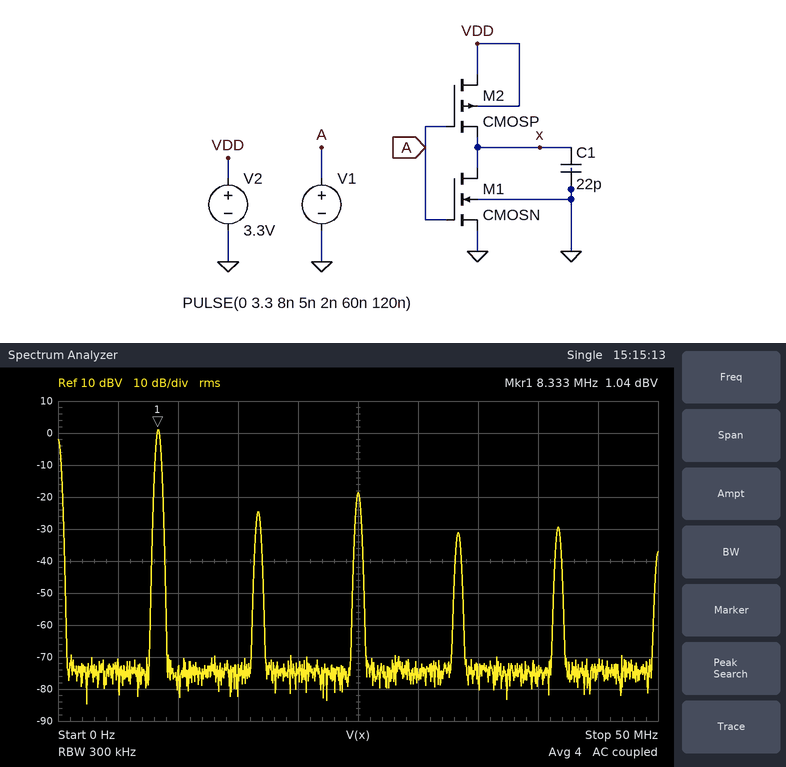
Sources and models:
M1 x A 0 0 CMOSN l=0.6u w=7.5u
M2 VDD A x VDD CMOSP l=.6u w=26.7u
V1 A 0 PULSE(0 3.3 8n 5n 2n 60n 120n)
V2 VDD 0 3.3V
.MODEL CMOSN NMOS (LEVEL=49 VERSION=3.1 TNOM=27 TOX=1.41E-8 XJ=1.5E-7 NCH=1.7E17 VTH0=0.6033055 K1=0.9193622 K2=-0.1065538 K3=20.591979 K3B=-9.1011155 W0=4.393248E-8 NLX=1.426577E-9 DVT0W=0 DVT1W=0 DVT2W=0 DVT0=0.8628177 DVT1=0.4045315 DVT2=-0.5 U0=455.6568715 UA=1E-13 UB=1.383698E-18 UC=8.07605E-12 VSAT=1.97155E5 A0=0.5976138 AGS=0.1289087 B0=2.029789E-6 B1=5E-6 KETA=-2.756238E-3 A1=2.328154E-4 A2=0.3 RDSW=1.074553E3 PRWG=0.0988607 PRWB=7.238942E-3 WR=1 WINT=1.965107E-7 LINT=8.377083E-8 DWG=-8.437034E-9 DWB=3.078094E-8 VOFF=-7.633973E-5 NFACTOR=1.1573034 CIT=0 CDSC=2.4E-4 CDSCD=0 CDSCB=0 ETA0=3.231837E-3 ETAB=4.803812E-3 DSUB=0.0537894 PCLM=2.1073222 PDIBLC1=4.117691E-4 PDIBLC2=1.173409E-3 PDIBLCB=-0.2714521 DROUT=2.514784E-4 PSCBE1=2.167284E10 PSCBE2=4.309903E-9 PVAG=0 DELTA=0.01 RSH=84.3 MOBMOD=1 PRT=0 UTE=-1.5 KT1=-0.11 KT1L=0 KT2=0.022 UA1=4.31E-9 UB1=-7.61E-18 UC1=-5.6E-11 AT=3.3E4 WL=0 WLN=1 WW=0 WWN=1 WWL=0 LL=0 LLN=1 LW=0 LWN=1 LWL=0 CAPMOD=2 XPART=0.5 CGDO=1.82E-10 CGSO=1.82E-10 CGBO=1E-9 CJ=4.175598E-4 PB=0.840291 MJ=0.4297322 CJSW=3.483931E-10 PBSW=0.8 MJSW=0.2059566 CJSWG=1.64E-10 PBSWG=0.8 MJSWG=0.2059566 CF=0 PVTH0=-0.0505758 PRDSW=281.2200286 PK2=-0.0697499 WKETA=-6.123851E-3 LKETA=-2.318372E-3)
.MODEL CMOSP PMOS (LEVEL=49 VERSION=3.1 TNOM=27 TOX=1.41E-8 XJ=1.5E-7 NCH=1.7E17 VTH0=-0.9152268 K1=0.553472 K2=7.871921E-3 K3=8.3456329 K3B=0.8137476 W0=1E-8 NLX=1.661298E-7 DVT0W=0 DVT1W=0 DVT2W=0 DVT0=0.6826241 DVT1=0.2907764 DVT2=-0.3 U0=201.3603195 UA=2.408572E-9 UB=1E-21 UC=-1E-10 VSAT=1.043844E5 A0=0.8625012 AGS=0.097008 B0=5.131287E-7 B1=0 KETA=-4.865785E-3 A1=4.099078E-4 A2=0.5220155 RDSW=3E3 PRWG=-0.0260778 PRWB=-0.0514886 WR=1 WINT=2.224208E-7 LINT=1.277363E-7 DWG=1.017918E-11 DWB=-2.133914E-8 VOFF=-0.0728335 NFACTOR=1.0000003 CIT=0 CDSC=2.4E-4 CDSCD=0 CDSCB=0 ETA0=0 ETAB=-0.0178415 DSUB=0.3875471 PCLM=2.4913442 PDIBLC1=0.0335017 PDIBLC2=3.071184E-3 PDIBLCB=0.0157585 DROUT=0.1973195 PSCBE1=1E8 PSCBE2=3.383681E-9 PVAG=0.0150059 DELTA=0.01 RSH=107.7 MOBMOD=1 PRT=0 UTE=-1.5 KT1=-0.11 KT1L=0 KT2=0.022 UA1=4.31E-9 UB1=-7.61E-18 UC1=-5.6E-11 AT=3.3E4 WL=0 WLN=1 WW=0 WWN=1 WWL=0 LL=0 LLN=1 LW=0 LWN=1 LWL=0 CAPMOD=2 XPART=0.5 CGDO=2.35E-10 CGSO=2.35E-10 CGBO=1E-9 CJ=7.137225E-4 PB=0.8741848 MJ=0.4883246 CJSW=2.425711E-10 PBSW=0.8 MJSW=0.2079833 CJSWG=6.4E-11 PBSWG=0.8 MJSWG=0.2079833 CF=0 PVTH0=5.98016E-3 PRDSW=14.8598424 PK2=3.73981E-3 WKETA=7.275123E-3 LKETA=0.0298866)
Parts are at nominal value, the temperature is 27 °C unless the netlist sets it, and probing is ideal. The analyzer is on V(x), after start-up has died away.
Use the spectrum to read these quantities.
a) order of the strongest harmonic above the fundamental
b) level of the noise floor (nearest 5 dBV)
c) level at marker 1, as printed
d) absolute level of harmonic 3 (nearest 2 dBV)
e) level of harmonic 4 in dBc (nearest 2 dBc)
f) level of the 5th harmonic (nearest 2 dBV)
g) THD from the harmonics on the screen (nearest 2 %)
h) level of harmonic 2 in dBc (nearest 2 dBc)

3
-75 dBV
1.04 dBV
-18 dBV
-32 dBc
-30 dBV
12 %
-26 dBc
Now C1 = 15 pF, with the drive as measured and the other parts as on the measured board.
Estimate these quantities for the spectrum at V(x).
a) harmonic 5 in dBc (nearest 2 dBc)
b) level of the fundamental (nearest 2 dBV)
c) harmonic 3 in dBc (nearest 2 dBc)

-28 dBc
2 dBV
-16 dBc
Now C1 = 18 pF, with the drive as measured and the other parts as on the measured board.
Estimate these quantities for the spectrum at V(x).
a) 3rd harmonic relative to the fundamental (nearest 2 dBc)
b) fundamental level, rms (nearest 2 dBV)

-18 dBc
2 dBV
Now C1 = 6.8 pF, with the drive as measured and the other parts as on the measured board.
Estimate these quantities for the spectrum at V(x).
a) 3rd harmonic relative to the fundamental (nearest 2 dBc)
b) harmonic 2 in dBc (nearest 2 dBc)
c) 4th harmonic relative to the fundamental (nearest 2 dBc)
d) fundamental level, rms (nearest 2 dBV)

-12 dBc
-28 dBc
-30 dBc
4 dBV
